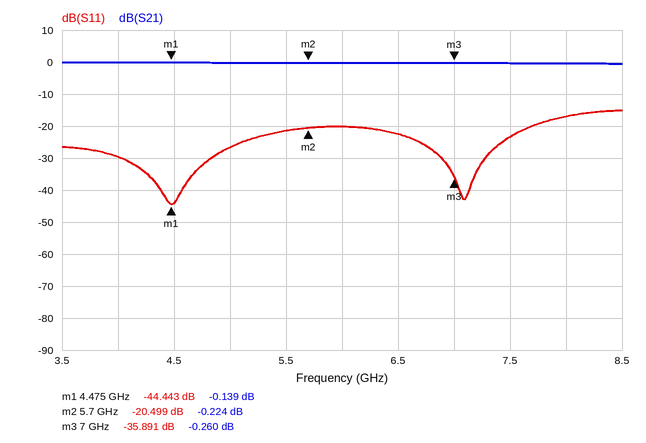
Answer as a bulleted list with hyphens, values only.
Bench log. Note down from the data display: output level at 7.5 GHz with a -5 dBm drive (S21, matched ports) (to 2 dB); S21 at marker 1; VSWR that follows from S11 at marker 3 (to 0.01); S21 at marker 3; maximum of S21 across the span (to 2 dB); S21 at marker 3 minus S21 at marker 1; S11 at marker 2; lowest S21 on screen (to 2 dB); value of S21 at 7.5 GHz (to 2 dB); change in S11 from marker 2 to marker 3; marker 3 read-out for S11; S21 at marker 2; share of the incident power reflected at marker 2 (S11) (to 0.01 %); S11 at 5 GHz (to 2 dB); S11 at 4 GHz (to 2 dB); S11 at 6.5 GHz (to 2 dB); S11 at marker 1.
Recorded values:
- -6 dBm
- -0.139 dB
- 1.03
- -0.260 dB
- 0 dB
- -0.121 dB
- -20.499 dB
- 0 dB
- 0 dB
- -15.392 dB
- -35.891 dB
- -0.224 dB
- 0.89 %
- -26 dB
- -30 dB
- -22 dB
- -44.443 dB
